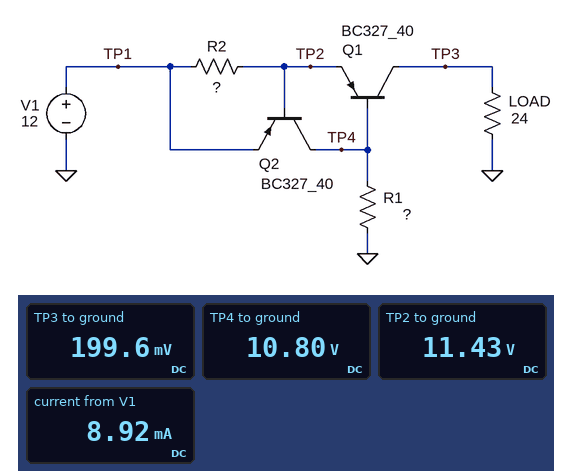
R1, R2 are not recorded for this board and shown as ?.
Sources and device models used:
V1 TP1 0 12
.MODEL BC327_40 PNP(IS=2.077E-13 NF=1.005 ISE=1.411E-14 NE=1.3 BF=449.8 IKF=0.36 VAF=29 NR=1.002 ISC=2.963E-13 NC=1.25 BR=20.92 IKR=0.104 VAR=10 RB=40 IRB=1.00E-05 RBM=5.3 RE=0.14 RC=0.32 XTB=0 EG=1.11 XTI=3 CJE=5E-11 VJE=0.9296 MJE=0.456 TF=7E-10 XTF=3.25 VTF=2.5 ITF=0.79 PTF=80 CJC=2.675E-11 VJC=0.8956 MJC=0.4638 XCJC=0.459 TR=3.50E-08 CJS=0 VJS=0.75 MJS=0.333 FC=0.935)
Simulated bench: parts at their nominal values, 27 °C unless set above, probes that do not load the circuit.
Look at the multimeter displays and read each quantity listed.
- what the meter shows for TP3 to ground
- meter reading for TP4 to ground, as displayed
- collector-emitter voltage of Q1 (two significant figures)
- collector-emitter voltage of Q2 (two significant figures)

199.6 mV
10.80 V
-11 V
-1.2 V
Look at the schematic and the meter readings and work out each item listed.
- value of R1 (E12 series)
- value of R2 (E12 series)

18 kΩ
68 Ω
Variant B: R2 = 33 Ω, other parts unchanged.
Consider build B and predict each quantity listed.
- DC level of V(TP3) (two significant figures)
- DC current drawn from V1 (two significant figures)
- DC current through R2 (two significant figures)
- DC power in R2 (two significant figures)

410 mV
18 mA
17 mA
9.7 mW
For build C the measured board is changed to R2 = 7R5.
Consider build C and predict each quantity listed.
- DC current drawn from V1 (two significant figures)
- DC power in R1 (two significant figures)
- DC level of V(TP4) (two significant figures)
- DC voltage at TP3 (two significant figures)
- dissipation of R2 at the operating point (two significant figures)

75 mA
6.4 mW
11 V
1.8 V
42 mW
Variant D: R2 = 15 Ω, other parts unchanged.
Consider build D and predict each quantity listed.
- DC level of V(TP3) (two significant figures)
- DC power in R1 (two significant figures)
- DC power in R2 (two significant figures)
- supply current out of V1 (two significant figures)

900 mV
6.4 mW
21 mW
38 mA
